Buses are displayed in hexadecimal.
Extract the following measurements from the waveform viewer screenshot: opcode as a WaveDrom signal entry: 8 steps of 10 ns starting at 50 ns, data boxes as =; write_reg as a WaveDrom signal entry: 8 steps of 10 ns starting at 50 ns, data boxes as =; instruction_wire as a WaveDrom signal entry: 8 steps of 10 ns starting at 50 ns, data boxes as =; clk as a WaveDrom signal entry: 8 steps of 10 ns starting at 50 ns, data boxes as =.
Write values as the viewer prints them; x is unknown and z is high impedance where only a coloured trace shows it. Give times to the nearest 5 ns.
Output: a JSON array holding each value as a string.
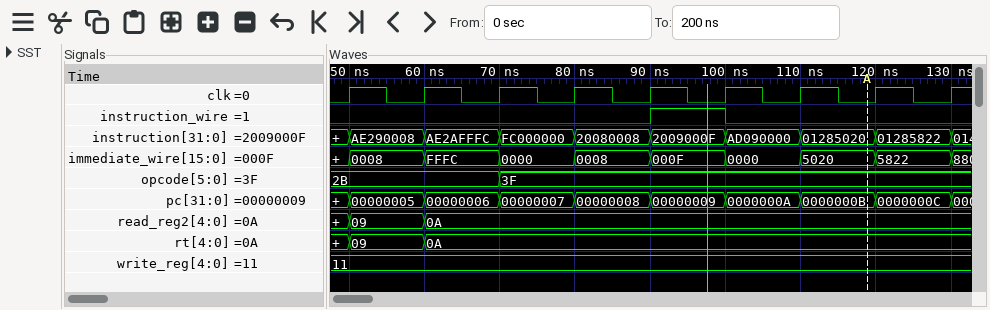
["{name: 'opcode', wave: '=.=.....', data: '2B 3F'}", "{name: 'write_reg', wave: '=.......', data: '11'}", "{name: 'instruction_wire', wave: '0...10..'}", "{name: 'clk', wave: 'p.......'}"]
